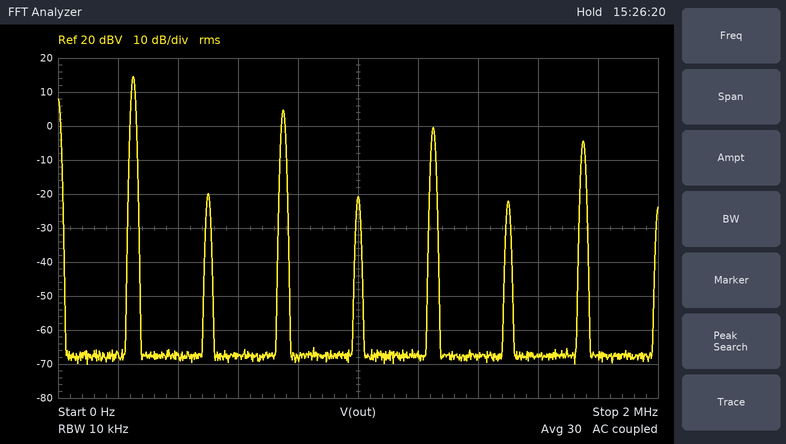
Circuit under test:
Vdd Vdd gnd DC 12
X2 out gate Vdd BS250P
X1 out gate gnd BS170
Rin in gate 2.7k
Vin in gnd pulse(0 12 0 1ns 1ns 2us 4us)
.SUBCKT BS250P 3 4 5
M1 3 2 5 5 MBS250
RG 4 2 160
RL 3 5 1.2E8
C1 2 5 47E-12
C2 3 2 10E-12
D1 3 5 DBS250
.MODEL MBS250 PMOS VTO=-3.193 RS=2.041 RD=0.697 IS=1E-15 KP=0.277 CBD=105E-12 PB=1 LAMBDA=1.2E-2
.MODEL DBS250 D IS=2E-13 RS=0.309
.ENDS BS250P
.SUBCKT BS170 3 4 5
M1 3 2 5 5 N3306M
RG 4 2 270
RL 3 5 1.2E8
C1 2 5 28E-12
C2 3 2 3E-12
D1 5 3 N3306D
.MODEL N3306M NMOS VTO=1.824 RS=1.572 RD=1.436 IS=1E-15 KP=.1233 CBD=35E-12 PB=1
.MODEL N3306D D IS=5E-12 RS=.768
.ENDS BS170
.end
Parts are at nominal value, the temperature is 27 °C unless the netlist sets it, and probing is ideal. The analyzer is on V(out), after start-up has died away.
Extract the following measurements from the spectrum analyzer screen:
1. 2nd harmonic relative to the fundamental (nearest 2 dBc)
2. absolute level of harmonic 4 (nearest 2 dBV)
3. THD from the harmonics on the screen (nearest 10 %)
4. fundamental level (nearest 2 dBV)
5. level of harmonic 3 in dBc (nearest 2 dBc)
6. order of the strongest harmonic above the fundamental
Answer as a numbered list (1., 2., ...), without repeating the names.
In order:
1. -34 dBc
2. -20 dBV
3. 40 %
4. 14 dBV
5. -10 dBc
6. 3
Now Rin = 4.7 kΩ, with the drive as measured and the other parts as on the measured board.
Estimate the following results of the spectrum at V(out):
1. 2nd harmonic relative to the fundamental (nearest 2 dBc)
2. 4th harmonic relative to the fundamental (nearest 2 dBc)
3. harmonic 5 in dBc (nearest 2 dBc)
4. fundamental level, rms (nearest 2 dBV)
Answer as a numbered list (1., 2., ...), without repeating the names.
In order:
1. -30 dBc
2. -32 dBc
3. -16 dBc
4. 14 dBV
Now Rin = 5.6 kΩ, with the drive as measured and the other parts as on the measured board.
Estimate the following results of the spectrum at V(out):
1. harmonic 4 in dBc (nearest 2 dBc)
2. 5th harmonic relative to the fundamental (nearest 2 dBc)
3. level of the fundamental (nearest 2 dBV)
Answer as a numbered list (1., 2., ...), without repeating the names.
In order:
1. -32 dBc
2. -18 dBc
3. 14 dBV
